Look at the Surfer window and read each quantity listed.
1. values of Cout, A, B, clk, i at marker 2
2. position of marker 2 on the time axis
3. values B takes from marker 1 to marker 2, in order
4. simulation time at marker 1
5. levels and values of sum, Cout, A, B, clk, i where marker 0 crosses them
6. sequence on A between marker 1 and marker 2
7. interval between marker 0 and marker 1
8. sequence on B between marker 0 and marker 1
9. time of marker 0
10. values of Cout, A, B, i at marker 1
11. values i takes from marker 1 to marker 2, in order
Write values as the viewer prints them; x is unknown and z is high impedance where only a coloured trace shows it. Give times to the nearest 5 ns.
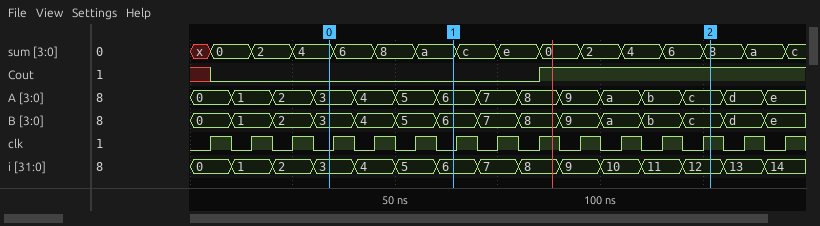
Cout=1, A=c, B=c, clk=1, i=12
125 ns
6, 7, 8, 9, a, b, c
65 ns
sum=4, Cout=0, A=3, B=3, clk=0, i=3
6, 7, 8, 9, a, b, c
30 ns
3, 4, 5, 6
35 ns
Cout=0, A=6, B=6, i=6
6, 7, 8, 9, 10, 11, 12
